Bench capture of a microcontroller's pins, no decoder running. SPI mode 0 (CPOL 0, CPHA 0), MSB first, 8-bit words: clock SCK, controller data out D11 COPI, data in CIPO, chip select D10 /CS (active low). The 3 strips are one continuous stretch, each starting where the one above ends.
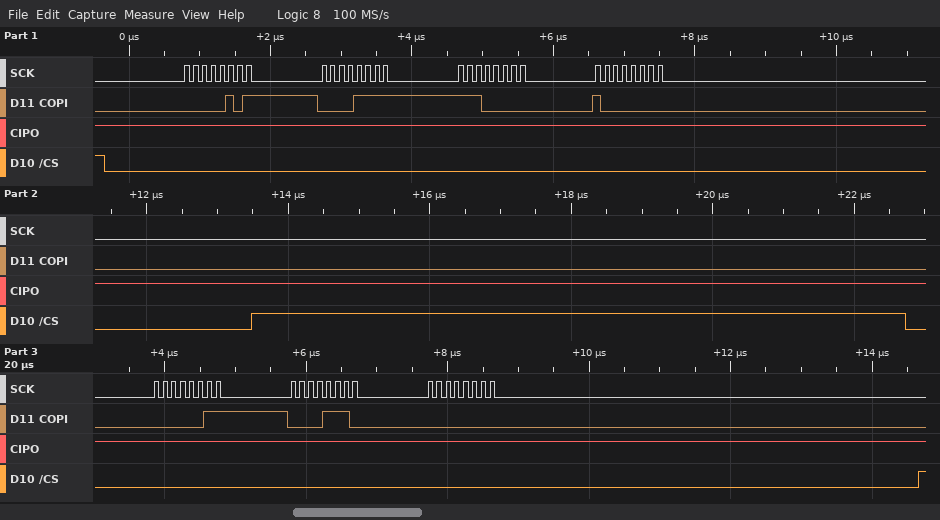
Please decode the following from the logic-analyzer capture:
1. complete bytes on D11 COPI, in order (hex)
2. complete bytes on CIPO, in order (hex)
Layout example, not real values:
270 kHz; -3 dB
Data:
05 0F E0 80 03 0E 00; FF FF FF FF FF FF FF
